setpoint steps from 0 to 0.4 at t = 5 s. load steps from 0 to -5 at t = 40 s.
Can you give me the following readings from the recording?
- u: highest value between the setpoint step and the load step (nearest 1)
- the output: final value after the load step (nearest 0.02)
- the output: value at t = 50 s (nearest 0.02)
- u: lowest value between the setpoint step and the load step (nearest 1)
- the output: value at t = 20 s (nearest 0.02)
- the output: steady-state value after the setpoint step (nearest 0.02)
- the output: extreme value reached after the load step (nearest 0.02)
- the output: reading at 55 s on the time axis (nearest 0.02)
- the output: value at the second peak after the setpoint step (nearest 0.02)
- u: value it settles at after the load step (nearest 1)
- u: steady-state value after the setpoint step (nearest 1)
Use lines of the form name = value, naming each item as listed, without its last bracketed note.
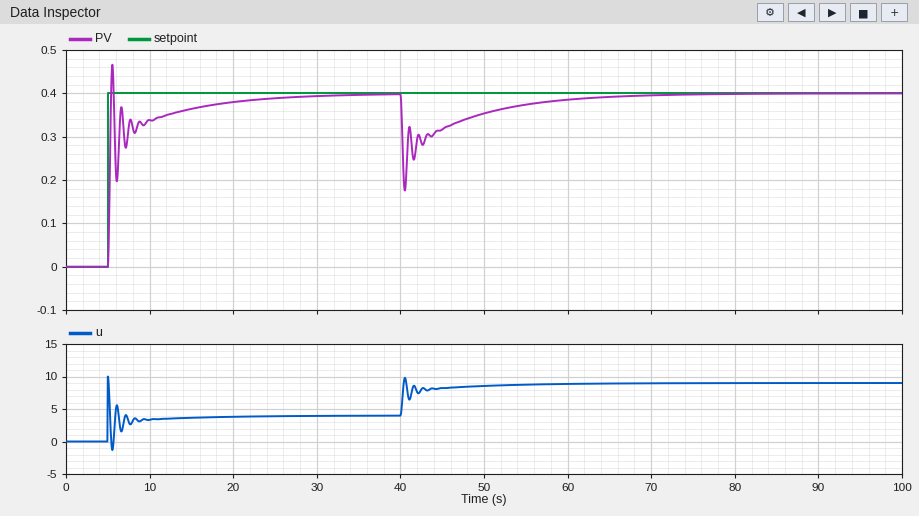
u: highest value between the setpoint step and the load step = 10
the output: final value after the load step = 0.40
the output: value at t = 50 s = 0.36
u: lowest value between the setpoint step and the load step = -1
the output: value at t = 20 s = 0.38
the output: steady-state value after the setpoint step = 0.40
the output: extreme value reached after the load step = 0.18
the output: reading at 55 s on the time axis = 0.38
the output: value at the second peak after the setpoint step = 0.36
u: value it settles at after the load step = 9
u: steady-state value after the setpoint step = 4
